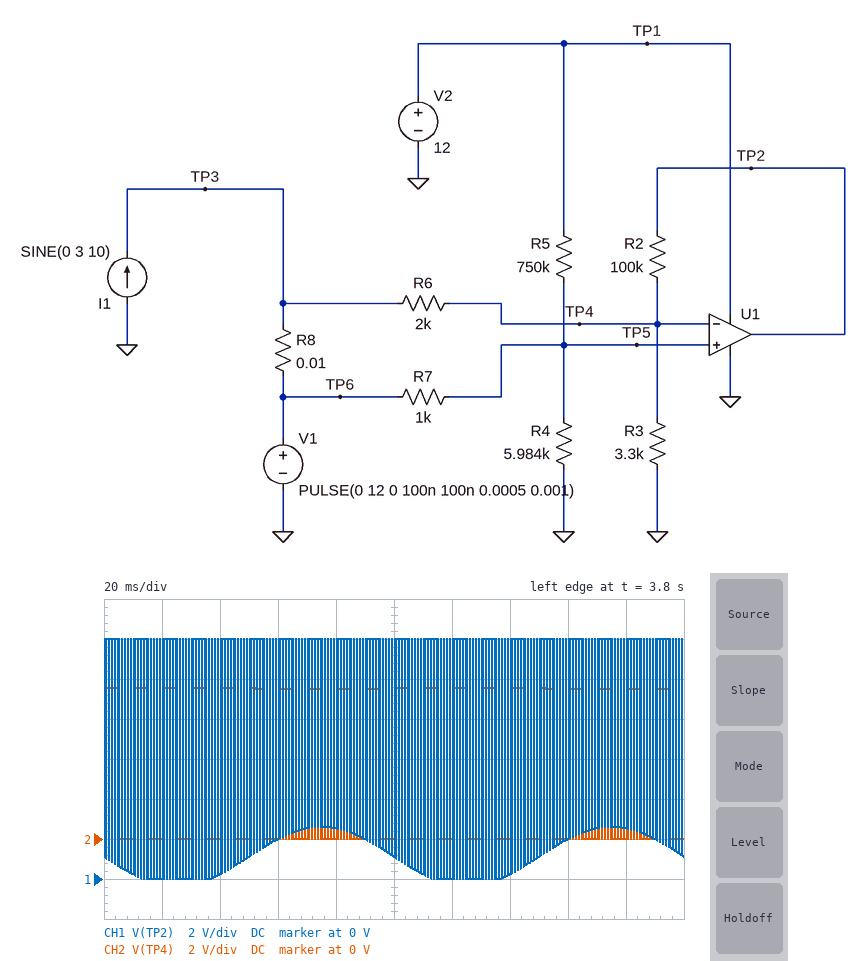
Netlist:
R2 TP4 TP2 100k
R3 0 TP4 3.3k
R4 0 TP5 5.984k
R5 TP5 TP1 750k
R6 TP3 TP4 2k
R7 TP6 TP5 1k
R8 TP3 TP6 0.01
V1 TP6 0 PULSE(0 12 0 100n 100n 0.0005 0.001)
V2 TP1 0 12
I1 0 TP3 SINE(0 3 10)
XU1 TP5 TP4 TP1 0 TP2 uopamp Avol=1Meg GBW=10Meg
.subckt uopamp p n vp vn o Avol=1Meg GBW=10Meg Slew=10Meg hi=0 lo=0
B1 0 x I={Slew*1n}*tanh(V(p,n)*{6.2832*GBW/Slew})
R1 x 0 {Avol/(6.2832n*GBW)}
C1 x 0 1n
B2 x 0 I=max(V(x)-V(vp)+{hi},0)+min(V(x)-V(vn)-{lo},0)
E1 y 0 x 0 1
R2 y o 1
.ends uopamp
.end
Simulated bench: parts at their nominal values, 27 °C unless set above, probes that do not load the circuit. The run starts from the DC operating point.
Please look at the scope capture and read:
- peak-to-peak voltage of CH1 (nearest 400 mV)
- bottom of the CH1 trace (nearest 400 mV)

12.0 V
0 V
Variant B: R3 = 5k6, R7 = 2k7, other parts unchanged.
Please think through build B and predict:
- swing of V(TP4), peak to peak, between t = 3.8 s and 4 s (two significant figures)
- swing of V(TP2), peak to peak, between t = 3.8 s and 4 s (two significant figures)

8.8 V
3.6 V
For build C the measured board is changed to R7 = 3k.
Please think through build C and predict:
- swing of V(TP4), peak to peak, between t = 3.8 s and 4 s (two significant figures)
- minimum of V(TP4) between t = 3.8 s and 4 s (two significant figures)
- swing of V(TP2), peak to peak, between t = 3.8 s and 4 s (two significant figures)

7.5 V
32 mV
11 V
